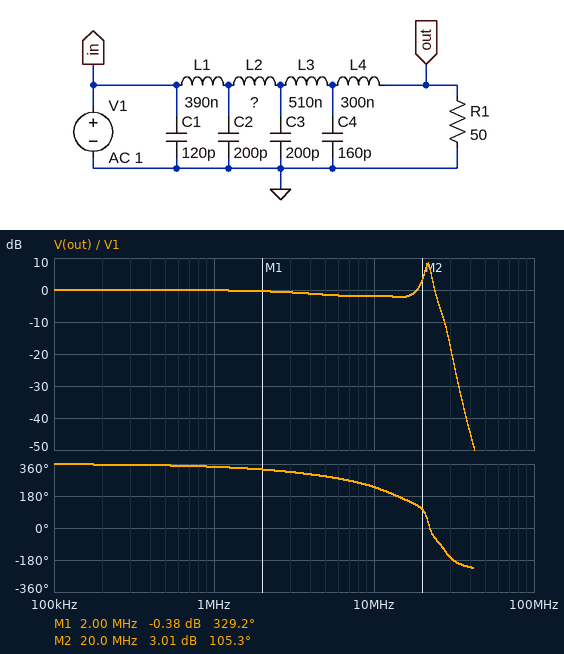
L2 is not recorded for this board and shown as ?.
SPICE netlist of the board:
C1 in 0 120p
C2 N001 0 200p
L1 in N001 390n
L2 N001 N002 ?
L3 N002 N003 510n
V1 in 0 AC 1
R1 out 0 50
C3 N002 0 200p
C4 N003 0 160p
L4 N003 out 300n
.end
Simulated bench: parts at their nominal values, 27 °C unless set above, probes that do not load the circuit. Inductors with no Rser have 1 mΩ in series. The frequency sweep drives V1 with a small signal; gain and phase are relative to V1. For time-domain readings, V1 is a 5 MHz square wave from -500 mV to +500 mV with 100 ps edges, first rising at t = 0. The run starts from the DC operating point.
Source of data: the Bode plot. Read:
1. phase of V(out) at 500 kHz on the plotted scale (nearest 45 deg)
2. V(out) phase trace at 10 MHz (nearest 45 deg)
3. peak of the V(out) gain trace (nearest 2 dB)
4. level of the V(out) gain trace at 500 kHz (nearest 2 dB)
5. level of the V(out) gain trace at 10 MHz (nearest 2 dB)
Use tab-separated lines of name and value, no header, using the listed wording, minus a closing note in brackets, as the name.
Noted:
phase of V(out) at 500 kHz on the plotted scale	360 deg
V(out) phase trace at 10 MHz	225 deg
peak of the V(out) gain trace	8 dB
level of the V(out) gain trace at 500 kHz	0 dB
level of the V(out) gain trace at 10 MHz	-2 dB
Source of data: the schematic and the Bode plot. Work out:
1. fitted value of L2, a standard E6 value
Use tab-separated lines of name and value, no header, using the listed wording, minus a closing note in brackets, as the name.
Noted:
fitted value of L2, a standard E6 value	1 µH
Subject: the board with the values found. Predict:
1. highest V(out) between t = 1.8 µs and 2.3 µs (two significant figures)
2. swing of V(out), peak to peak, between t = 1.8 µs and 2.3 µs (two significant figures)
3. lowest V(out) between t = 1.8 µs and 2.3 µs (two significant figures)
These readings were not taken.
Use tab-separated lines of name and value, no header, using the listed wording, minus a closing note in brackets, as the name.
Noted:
highest V(out) between t = 1.8 µs and 2.3 µs	560 mV
swing of V(out), peak to peak, between t = 1.8 µs and 2.3 µs	1.1 V
lowest V(out) between t = 1.8 µs and 2.3 µs	-560 mV
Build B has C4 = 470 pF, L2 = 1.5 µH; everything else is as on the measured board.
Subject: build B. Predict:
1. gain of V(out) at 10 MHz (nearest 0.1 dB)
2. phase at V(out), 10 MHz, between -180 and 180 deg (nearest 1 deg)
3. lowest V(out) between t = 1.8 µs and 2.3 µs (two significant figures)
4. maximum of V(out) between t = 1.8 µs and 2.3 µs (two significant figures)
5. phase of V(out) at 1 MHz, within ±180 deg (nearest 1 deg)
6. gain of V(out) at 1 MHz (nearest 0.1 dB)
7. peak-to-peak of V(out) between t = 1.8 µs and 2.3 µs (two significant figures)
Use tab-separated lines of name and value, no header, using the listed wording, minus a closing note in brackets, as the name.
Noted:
gain of V(out) at 10 MHz	-8.7 dB
phase at V(out), 10 MHz, between -180 and 180 deg	-169 deg
lowest V(out) between t = 1.8 µs and 2.3 µs	-580 mV
maximum of V(out) between t = 1.8 µs and 2.3 µs	580 mV
phase of V(out) at 1 MHz, within ±180 deg	-20 deg
gain of V(out) at 1 MHz	0 dB
peak-to-peak of V(out) between t = 1.8 µs and 2.3 µs	1.2 V
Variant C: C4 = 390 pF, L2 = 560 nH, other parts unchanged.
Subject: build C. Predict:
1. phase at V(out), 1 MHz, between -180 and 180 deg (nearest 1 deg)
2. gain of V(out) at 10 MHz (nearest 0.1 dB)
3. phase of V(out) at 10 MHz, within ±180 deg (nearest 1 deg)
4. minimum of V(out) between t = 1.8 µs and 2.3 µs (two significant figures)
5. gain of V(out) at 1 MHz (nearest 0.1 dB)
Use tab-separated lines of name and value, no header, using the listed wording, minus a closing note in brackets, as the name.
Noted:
phase at V(out), 1 MHz, between -180 and 180 deg	-13 deg
gain of V(out) at 10 MHz	-2.4 dB
phase of V(out) at 10 MHz, within ±180 deg	-154 deg
minimum of V(out) between t = 1.8 µs and 2.3 µs	-670 mV
gain of V(out) at 1 MHz	0.1 dB
